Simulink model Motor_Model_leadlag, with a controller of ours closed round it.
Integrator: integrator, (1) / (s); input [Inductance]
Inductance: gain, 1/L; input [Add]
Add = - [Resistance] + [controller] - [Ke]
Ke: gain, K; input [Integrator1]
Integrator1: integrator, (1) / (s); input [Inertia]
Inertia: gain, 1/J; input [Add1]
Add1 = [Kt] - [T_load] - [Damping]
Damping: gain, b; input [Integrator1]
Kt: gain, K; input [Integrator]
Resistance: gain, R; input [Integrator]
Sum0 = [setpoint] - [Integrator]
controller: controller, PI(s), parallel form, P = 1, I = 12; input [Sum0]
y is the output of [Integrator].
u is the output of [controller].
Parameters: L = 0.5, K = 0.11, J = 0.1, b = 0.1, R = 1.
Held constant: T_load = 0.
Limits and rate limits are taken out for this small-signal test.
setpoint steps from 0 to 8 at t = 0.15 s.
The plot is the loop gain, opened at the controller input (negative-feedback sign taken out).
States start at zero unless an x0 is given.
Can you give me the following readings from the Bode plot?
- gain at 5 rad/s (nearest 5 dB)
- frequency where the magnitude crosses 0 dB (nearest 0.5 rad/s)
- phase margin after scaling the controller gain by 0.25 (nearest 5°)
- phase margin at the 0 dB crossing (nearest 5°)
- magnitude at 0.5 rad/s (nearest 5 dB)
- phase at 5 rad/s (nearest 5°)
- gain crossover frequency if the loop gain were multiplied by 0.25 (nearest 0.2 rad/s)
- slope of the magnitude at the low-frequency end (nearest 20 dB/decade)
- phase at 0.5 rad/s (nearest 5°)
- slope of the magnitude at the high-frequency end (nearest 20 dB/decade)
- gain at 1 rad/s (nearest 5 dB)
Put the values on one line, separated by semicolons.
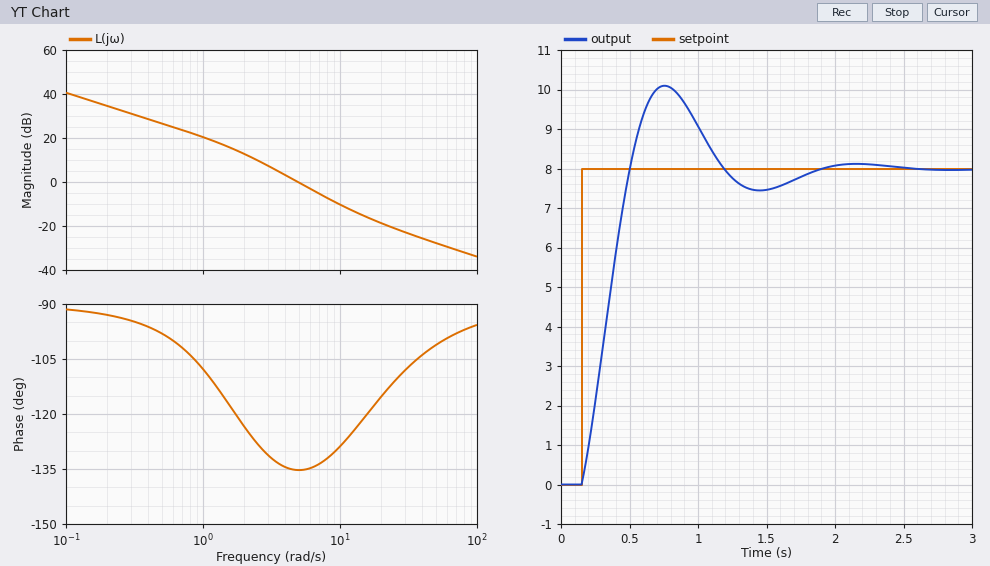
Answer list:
0 dB; 5.0 rad/s; 55°; 45°; 25 dB; -135°; 2.2 rad/s; -20 dB/decade; -100°; -20 dB/decade; 20 dB
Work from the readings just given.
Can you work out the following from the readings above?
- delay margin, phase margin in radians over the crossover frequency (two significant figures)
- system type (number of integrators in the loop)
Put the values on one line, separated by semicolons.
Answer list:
0.16 s; 1
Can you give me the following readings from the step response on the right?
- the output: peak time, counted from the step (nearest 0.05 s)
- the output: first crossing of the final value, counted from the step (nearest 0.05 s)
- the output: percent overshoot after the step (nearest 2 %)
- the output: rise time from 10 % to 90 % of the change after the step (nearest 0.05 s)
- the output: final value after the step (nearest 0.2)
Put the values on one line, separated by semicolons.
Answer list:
0.60 s; 0.35 s; 26 %; 0.25 s; 8.0
